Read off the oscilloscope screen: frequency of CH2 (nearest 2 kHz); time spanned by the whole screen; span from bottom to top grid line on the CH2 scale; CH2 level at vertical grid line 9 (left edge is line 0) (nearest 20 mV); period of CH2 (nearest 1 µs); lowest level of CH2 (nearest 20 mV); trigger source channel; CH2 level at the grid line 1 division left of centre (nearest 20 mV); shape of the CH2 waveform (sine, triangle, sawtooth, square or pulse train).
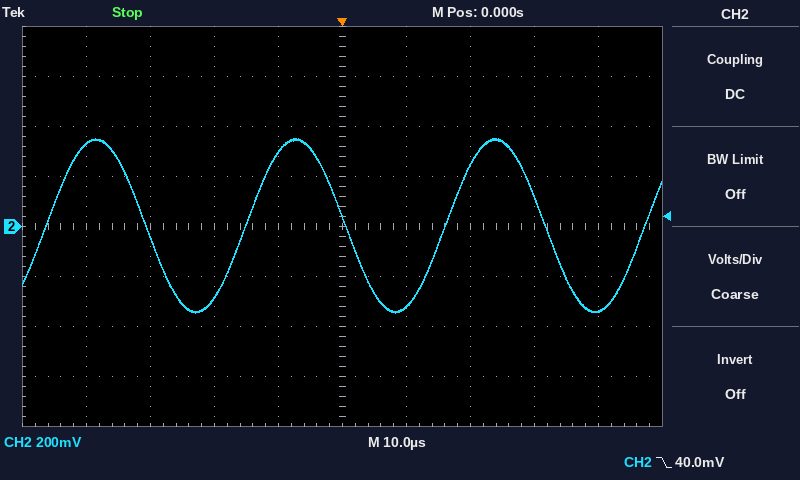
32 kHz
100 µs
1.6 V
-340 mV
31 µs
-340 mV
CH2
300 mV
sine
